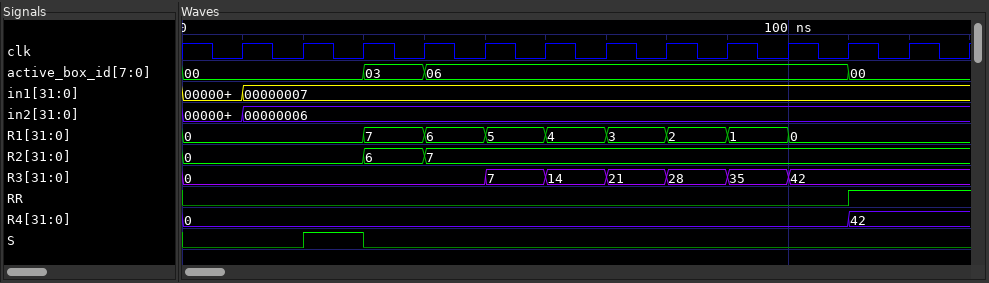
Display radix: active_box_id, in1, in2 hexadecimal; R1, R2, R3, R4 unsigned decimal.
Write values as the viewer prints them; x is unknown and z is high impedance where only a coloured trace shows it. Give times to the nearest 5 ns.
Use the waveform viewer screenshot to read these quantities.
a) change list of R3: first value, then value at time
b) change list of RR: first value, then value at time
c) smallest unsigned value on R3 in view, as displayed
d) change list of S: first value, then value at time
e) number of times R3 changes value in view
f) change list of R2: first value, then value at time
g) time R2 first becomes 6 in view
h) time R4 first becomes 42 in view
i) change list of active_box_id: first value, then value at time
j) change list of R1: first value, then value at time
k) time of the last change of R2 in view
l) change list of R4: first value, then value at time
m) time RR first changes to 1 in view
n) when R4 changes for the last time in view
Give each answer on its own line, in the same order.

0, 7 at 50 ns, 14 at 60 ns, 21 at 70 ns, 28 at 80 ns, 35 at 90 ns, 42 at 100 ns
0, 1 at 110 ns
0
0, 1 at 20 ns, 0 at 30 ns
6
0, 6 at 30 ns, 7 at 40 ns
30 ns
110 ns
00, 03 at 30 ns, 06 at 40 ns, 00 at 110 ns
0, 7 at 30 ns, 6 at 40 ns, 5 at 50 ns, 4 at 60 ns, 3 at 70 ns, 2 at 80 ns, 1 at 90 ns, 0 at 100 ns
40 ns
0, 42 at 110 ns
110 ns
110 ns
